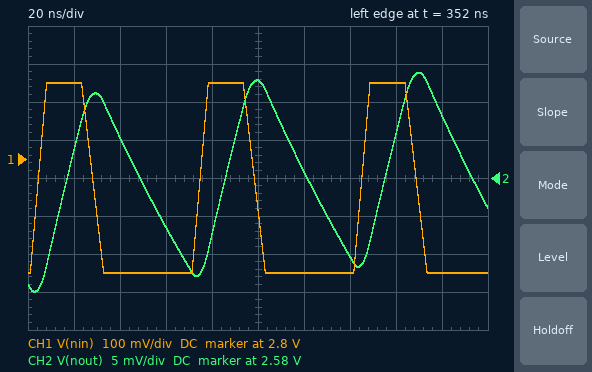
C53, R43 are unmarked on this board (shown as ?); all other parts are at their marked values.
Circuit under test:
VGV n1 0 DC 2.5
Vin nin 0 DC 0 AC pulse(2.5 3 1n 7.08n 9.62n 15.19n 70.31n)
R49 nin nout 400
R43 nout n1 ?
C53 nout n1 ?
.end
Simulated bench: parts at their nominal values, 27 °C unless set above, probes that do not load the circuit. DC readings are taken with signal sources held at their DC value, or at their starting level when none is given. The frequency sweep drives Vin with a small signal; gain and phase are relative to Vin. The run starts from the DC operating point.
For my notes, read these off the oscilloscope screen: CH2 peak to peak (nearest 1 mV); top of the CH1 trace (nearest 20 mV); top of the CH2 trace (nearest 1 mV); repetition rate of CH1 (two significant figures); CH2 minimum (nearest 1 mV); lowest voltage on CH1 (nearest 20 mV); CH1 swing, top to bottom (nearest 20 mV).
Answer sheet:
29 mV
3.00 V
2.594 V
14 MHz
2.565 V
2.50 V
500 mV
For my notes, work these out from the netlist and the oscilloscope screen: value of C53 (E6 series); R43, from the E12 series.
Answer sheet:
680 pF
390 Ω
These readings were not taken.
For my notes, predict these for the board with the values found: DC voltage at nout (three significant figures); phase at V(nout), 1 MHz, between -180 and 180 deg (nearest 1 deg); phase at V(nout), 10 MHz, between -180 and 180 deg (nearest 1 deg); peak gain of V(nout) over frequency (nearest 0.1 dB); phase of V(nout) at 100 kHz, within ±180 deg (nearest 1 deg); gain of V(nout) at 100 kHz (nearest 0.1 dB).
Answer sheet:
1.27 V
-40 deg
-83 deg
-6.1 dB
-5 deg
-6.2 dB
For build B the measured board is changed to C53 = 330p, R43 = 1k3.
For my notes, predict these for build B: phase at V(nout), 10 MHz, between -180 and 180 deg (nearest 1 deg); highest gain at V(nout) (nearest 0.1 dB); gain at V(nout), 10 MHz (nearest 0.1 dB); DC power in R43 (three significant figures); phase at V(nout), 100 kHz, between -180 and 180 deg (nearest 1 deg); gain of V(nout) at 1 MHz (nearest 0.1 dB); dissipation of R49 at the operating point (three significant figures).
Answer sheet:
-81 deg
-2.3 dB
-18.5 dB
2.81 mW
-4 deg
-3.8 dB
865 µW
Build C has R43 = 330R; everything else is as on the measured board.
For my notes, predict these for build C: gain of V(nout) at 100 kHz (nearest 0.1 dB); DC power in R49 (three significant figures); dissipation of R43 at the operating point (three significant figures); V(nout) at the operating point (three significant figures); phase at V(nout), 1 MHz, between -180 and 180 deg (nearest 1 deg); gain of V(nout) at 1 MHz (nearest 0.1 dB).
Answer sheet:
-6.9 dB
4.69 mW
3.87 mW
1.37 V
-38 deg
-8.9 dB
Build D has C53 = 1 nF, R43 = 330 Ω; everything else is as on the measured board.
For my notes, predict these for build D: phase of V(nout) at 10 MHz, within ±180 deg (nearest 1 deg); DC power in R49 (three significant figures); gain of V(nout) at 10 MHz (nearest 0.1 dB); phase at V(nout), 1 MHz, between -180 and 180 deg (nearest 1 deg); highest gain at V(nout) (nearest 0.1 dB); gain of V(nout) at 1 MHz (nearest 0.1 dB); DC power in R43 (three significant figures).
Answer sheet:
-85 deg
4.69 mW
-28.0 dB
-49 deg
-6.9 dB
-10.5 dB
3.87 mW
